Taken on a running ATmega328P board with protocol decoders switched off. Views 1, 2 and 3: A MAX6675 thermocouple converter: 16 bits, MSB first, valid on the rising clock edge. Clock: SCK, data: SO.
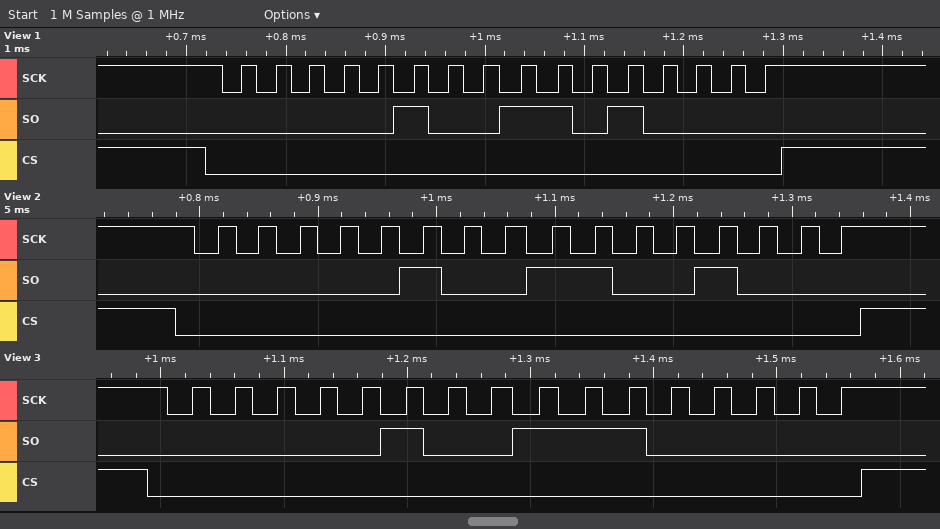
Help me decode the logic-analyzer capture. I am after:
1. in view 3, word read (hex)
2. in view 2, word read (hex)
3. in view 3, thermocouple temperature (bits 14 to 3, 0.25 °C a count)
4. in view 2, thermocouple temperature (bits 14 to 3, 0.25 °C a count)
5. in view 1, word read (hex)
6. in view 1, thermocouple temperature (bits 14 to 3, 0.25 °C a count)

0x04E0
0x04C8
39.00 °C
38.25 °C
0x04D0
38.50 °C
